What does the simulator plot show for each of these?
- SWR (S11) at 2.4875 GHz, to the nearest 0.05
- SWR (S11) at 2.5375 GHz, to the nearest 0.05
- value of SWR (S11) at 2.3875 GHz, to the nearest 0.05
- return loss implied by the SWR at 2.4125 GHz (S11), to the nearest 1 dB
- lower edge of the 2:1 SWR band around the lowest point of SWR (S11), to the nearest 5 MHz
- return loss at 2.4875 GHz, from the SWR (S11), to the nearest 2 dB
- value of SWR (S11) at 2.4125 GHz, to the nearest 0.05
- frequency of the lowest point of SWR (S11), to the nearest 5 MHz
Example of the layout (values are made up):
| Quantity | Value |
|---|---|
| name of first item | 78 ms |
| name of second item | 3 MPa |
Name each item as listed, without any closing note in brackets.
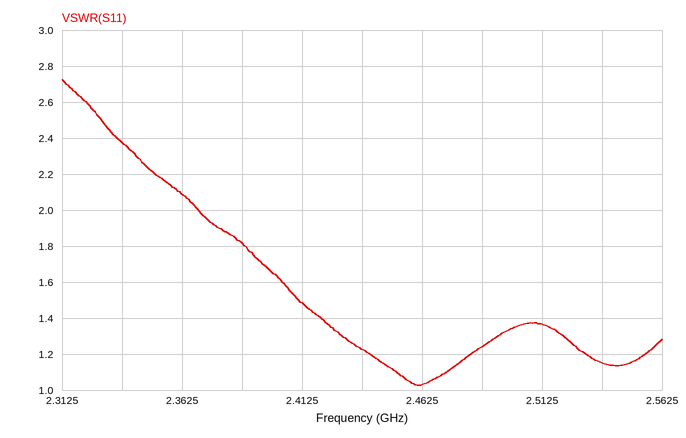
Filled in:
| Quantity | Value |
|---|---|
| SWR (S11) at 2.4875 GHz, to the nearest 0.05 | 1.25 |
| SWR (S11) at 2.5375 GHz, to the nearest 0.05 | 1.15 |
| value of SWR (S11) at 2.3875 GHz, to the nearest 0.05 | 1.80 |
| return loss implied by the SWR at 2.4125 GHz (S11), to the nearest 1 dB | 14 dB |
| lower edge of the 2:1 SWR band around the lowest point of SWR (S11), to the nearest 5 MHz | 2.370 GHz |
| return loss at 2.4875 GHz, from the SWR (S11), to the nearest 2 dB | 20 dB |
| value of SWR (S11) at 2.4125 GHz, to the nearest 0.05 | 1.50 |
| frequency of the lowest point of SWR (S11), to the nearest 5 MHz | 2.460 GHz |
